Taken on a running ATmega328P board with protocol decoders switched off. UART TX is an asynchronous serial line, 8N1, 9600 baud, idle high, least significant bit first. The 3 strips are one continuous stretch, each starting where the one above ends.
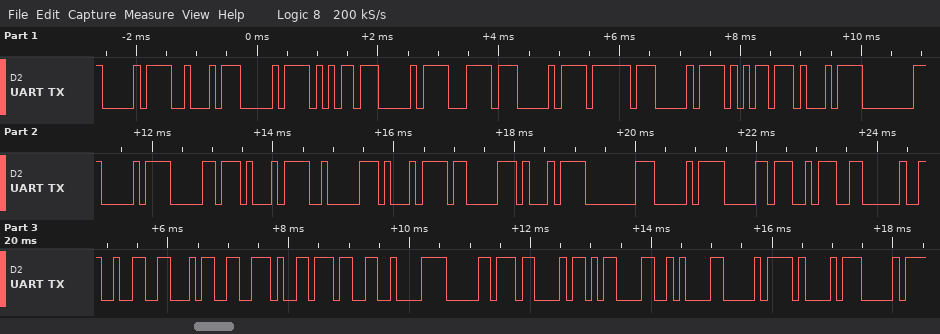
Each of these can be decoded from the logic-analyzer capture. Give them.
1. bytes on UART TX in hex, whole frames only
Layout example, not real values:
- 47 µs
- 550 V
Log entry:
- D0 A2 D0 B5 D0 BC D0 BF D0 B5 D1 80 D0 B0 D1 82 D1 83 D1 80 D0 B0 3A 20 32 34 2E 37 C2 B0 43 0D 0A D0 A1 D0
